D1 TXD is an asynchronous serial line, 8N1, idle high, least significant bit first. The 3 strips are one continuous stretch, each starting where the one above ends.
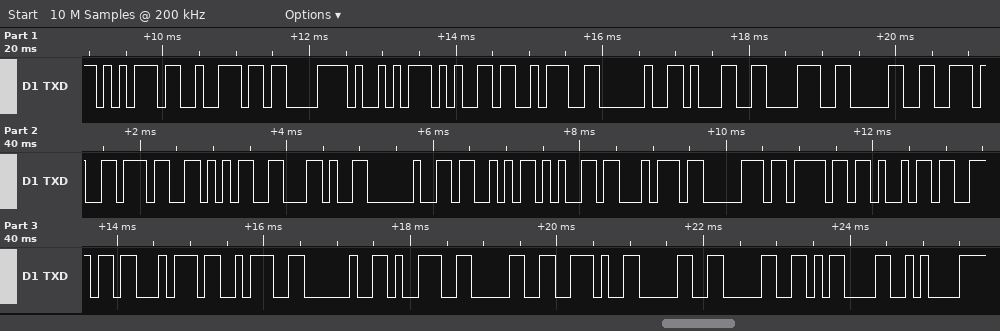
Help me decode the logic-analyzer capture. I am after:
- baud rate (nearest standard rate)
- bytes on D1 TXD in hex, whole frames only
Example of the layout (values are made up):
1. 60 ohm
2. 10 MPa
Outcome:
1. 9600 baud
2. 75 72 C3 A9 65 3A 20 31 38 30 2E 37 35 2C 20 53 65 74 70 6F 69 6E 74 3A 20 39 30 2E 30 30 0D 0A
